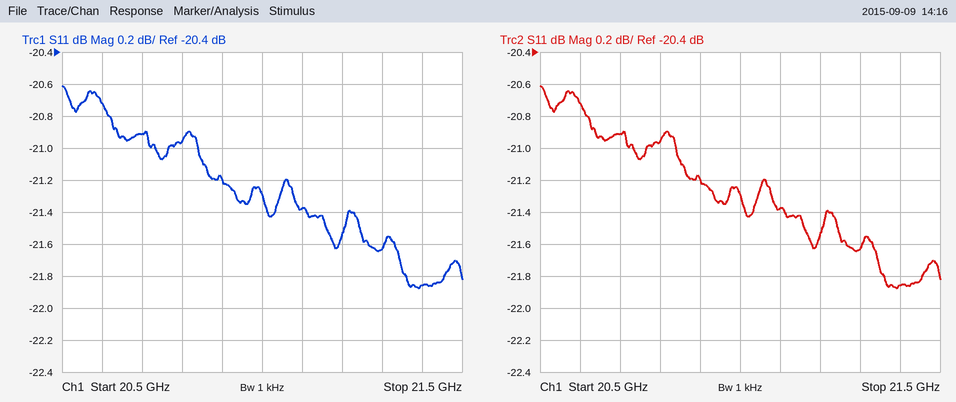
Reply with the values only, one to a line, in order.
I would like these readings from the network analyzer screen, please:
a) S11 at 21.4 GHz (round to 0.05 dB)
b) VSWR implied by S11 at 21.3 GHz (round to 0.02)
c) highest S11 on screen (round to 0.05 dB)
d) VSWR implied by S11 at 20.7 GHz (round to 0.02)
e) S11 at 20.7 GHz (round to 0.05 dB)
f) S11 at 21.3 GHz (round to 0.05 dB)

-21.85 dB
1.18
-20.60 dB
1.20
-20.90 dB
-21.65 dB
